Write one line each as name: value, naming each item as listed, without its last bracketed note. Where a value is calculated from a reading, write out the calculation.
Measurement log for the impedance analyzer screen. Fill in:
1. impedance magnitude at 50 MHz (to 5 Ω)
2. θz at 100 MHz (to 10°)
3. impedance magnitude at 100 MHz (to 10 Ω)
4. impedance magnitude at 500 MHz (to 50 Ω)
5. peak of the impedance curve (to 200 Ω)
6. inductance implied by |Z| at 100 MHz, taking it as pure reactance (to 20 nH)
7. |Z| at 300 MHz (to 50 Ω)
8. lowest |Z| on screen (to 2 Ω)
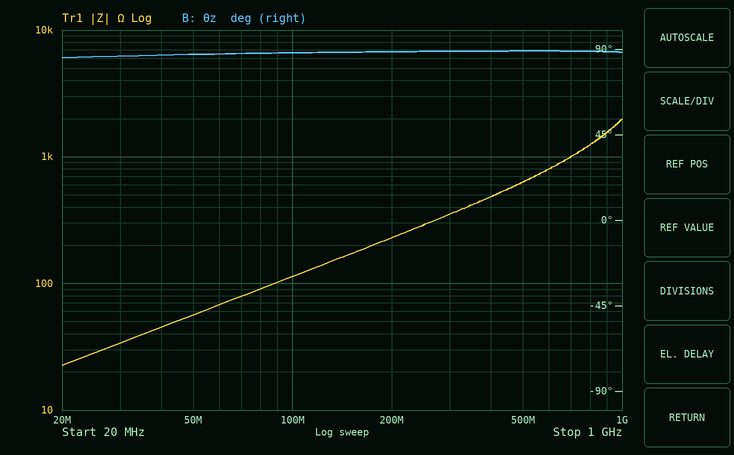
impedance magnitude at 50 MHz: 55 Ω
θz at 100 MHz: 90°
impedance magnitude at 100 MHz: 110 Ω
impedance magnitude at 500 MHz: 650 Ω
peak of the impedance curve: 2.0 kΩ
inductance implied by |Z| at 100 MHz, taking it as pure reactance: L = 110 Ω/(2π × 100 MHz) ≈ 175 nH, so 180 nH to the nearest 20 nH
|Z| at 300 MHz: 350 Ω
lowest |Z| on screen: 22 Ω
